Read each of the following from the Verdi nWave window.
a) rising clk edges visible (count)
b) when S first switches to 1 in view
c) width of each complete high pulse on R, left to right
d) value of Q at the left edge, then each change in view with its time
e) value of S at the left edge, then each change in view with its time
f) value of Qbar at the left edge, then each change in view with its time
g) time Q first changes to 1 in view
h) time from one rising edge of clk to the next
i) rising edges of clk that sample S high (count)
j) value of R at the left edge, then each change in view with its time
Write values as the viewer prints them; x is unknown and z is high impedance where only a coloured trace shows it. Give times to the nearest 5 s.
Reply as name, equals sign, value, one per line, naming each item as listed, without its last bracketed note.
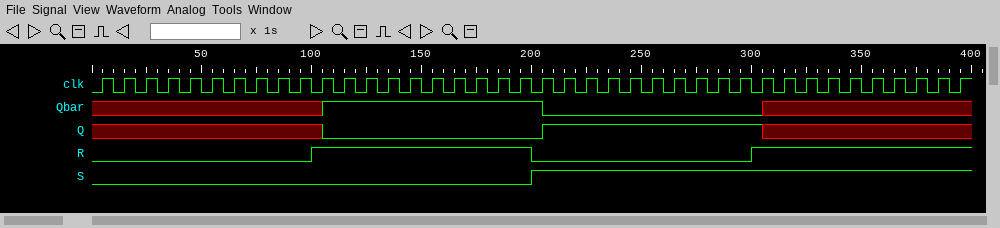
rising clk edges visible = 40
when S first switches to 1 in view = 200 s
width of each complete high pulse on R, left to right = 100 s
value of Q at the left edge, then each change in view with its time = x, 0 at 105 s, 1 at 205 s, x at 305 s
value of S at the left edge, then each change in view with its time = 0, 1 at 200 s
value of Qbar at the left edge, then each change in view with its time = x, 1 at 105 s, 0 at 205 s, x at 305 s
time Q first changes to 1 in view = 205 s
time from one rising edge of clk to the next = 10 s
rising edges of clk that sample S high = 20
value of R at the left edge, then each change in view with its time = 0, 1 at 100 s, 0 at 200 s, 1 at 300 s
